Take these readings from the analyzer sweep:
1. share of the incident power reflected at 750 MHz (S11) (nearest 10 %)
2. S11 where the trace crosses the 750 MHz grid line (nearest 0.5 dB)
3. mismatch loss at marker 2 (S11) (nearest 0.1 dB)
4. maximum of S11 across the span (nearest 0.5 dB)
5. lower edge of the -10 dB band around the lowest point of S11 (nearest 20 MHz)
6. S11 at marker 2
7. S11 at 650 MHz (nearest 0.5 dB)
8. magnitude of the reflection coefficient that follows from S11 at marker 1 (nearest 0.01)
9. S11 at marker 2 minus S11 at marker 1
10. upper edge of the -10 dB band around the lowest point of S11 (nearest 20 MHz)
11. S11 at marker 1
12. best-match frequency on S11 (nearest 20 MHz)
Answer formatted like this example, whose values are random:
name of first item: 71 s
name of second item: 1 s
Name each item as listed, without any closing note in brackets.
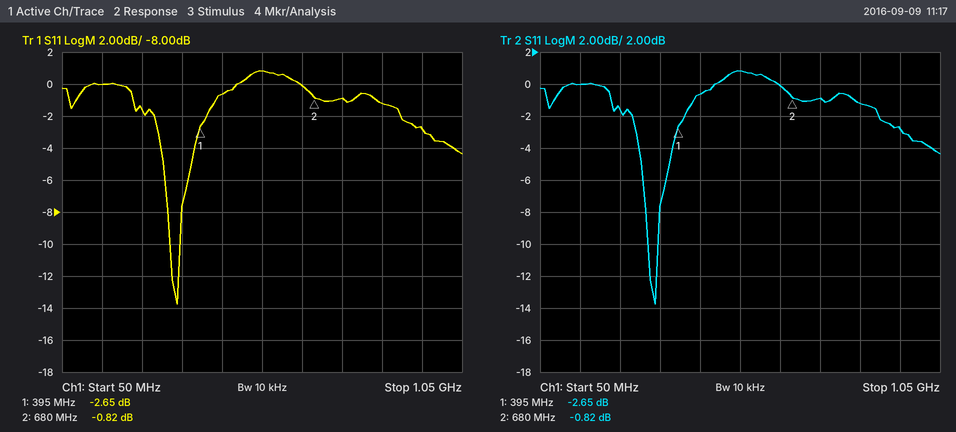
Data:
share of the incident power reflected at 750 MHz (S11): 80 %
S11 where the trace crosses the 750 MHz grid line: -1.0 dB
mismatch loss at marker 2 (S11): 7.6 dB
maximum of S11 across the span: 1.0 dB
lower edge of the -10 dB band around the lowest point of S11: 320 MHz
S11 at marker 2: -0.82 dB
S11 at 650 MHz: 0.0 dB
magnitude of the reflection coefficient that follows from S11 at marker 1: 0.74
S11 at marker 2 minus S11 at marker 1: 1.83 dB
upper edge of the -10 dB band around the lowest point of S11: 340 MHz
S11 at marker 1: -2.65 dB
best-match frequency on S11: 340 MHz
